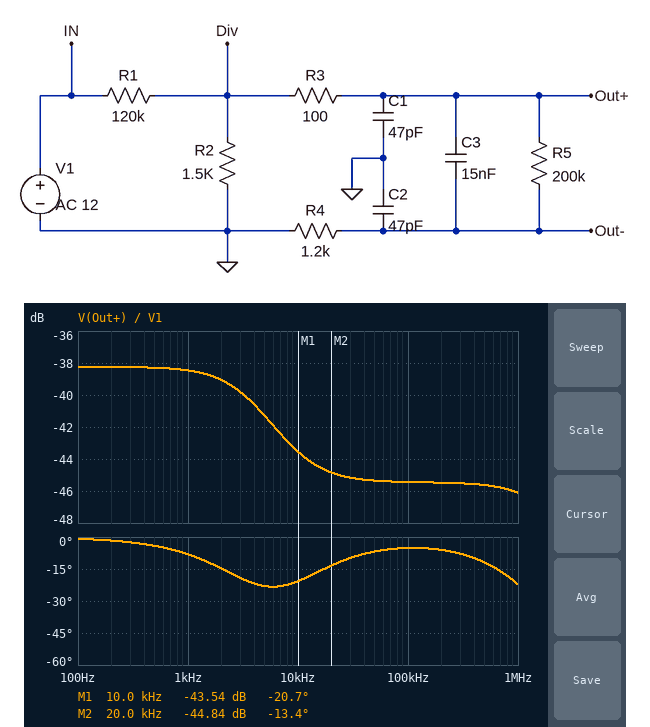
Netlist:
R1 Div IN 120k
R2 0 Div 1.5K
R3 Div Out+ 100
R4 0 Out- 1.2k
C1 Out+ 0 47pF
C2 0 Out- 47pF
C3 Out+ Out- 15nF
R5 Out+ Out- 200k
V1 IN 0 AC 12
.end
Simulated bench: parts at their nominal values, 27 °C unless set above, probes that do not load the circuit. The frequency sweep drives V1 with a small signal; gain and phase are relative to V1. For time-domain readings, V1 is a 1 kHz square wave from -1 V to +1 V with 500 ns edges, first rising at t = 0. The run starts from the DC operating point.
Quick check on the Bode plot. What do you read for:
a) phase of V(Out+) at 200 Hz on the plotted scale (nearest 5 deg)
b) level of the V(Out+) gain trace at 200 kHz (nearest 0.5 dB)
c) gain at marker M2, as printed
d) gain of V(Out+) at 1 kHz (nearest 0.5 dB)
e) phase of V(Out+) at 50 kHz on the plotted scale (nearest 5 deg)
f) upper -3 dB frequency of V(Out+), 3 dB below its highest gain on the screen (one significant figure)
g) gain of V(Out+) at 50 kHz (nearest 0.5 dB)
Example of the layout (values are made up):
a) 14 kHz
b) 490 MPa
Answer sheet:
a) 0 deg
b) -45.5 dB
c) -44.84 dB
d) -38.5 dB
e) -5 deg
f) 5 kHz
g) -45.5 dB
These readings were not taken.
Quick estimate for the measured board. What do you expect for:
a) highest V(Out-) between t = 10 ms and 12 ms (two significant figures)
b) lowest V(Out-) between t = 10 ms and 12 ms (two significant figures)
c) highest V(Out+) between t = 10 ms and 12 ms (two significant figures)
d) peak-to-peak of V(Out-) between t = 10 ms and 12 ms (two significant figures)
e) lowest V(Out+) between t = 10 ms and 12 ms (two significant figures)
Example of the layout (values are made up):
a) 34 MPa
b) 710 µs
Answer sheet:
a) 10 mV
b) -10 mV
c) 12 mV
d) 21 mV
e) -12 mV
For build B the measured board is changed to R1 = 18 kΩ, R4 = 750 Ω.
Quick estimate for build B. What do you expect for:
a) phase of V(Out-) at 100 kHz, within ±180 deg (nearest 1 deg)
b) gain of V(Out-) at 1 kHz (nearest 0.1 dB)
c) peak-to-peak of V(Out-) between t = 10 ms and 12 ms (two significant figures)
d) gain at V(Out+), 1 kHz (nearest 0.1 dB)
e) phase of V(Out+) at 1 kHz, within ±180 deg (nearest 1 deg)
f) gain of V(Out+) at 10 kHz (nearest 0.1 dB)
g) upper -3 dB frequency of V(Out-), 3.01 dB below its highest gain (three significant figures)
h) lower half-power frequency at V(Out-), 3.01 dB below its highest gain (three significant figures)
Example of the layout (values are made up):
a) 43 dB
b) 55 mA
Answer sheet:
a) 1 deg
b) -45.6 dB
c) 100 mV
d) -22.5 dB
e) -8 deg
f) -27.9 dB
g) 3.41 MHz
h) 4.78 kHz
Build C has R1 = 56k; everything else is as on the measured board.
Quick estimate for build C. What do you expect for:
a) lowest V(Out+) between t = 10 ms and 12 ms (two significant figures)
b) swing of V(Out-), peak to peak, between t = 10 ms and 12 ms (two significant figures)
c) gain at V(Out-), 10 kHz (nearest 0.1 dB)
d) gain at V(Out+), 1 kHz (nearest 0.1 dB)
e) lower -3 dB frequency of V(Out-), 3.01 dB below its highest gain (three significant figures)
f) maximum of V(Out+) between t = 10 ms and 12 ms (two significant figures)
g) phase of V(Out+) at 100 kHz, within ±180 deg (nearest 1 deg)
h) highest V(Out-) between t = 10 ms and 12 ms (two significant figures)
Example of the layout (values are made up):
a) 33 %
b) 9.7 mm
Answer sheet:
a) -26 mV
b) 44 mV
c) -39.5 dB
d) -32.0 dB
e) 3.88 kHz
f) 26 mV
g) -5 deg
h) 22 mV
